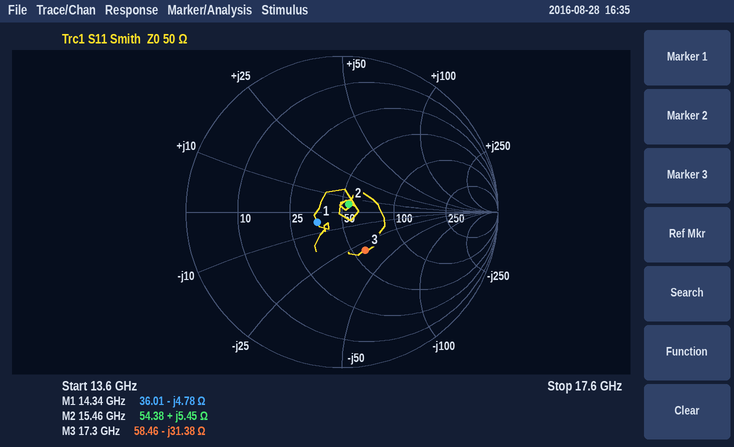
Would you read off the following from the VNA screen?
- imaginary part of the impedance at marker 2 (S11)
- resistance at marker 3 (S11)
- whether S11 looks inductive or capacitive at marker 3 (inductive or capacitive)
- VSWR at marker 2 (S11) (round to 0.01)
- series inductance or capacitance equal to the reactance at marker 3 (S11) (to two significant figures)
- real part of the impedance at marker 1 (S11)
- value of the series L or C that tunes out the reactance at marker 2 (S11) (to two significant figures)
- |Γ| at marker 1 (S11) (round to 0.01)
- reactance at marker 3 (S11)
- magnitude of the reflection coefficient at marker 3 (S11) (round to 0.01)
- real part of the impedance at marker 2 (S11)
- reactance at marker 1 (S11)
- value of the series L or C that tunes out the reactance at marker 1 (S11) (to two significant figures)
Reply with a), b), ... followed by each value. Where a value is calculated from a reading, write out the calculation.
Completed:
a) +5.45 Ω
b) 58.46 Ω
c) capacitive
d) 1.14
e) C = 1/(2π × 17.3 GHz × 31.38 Ω) ≈ 293 fF, so 290 fF to two significant figures
f) 36.01 Ω
g) C = 1/(2π × 15.46 GHz × 5.45 Ω) ≈ 1.9 pF
h) 0.17
i) -31.38 Ω
j) 0.29
k) 54.38 Ω
l) -4.78 Ω
m) L = 4.78 Ω/(2π × 14.34 GHz) ≈ 53 pH
